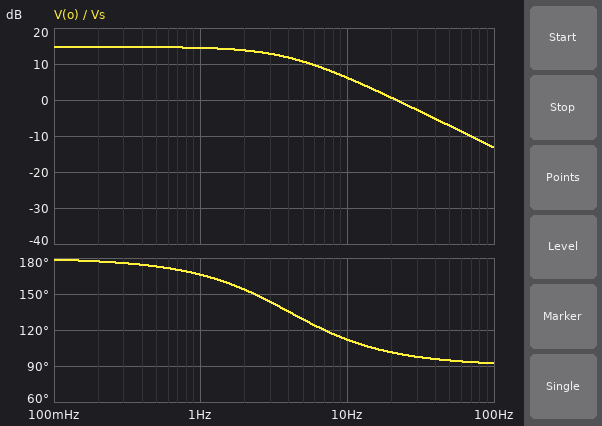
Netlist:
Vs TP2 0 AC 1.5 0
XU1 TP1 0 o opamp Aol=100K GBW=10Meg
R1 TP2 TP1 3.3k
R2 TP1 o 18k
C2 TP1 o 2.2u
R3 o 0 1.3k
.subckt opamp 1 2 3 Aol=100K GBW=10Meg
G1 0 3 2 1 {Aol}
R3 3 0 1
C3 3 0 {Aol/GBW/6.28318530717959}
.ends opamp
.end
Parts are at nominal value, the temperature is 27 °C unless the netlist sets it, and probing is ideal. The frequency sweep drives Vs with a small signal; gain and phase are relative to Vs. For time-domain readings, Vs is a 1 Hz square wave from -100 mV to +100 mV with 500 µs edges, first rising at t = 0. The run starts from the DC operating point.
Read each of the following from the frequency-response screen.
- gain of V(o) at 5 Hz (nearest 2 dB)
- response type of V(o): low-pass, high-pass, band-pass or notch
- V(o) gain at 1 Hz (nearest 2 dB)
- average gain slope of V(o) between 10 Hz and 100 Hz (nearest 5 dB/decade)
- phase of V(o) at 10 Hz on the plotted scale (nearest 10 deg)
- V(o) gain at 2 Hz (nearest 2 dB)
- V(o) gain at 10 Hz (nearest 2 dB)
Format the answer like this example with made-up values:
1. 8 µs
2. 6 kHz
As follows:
1. 10 dB
2. low-pass
3. 14 dB
4. -20 dB/decade
5. 110 deg
6. 14 dB
7. 6 dB
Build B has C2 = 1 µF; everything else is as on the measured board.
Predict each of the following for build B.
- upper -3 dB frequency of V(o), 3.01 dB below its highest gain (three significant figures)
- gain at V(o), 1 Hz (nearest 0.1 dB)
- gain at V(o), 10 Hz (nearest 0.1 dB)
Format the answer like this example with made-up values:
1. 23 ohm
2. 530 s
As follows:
1. 8.84 Hz
2. 14.7 dB
3. 11.2 dB
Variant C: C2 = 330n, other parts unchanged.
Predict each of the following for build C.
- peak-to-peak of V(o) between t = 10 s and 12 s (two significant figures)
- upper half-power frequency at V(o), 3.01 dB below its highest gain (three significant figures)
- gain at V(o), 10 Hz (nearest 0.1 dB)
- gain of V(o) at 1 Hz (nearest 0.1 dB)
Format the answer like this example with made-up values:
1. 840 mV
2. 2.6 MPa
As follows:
1. 1.1 V
2. 26.8 Hz
3. 14.2 dB
4. 14.7 dB
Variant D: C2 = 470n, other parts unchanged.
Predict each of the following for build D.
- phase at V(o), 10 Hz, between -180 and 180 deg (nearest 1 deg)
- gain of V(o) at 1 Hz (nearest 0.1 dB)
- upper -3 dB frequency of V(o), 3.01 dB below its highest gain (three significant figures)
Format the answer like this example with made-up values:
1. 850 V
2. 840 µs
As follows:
1. 152 deg
2. 14.7 dB
3. 18.8 Hz
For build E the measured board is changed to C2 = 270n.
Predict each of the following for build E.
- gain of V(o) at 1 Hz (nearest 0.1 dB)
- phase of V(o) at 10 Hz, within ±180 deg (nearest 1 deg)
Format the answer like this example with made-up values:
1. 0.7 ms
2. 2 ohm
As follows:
1. 14.7 dB
2. 163 deg
